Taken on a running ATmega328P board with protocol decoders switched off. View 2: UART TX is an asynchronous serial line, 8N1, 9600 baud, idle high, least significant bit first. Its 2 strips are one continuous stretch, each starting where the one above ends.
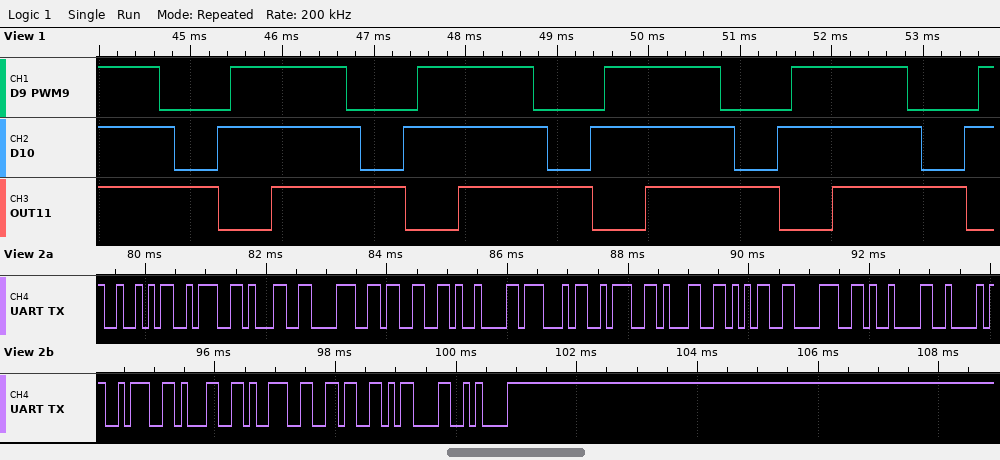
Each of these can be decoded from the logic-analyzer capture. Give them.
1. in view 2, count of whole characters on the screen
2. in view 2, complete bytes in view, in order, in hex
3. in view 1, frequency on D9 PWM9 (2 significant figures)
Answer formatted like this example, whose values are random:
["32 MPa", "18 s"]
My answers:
["19", "52 3A 31 38 33 09 47 3A 31 35 38 09 42 3A 31 39 36 0D 0A", "490 Hz"]
